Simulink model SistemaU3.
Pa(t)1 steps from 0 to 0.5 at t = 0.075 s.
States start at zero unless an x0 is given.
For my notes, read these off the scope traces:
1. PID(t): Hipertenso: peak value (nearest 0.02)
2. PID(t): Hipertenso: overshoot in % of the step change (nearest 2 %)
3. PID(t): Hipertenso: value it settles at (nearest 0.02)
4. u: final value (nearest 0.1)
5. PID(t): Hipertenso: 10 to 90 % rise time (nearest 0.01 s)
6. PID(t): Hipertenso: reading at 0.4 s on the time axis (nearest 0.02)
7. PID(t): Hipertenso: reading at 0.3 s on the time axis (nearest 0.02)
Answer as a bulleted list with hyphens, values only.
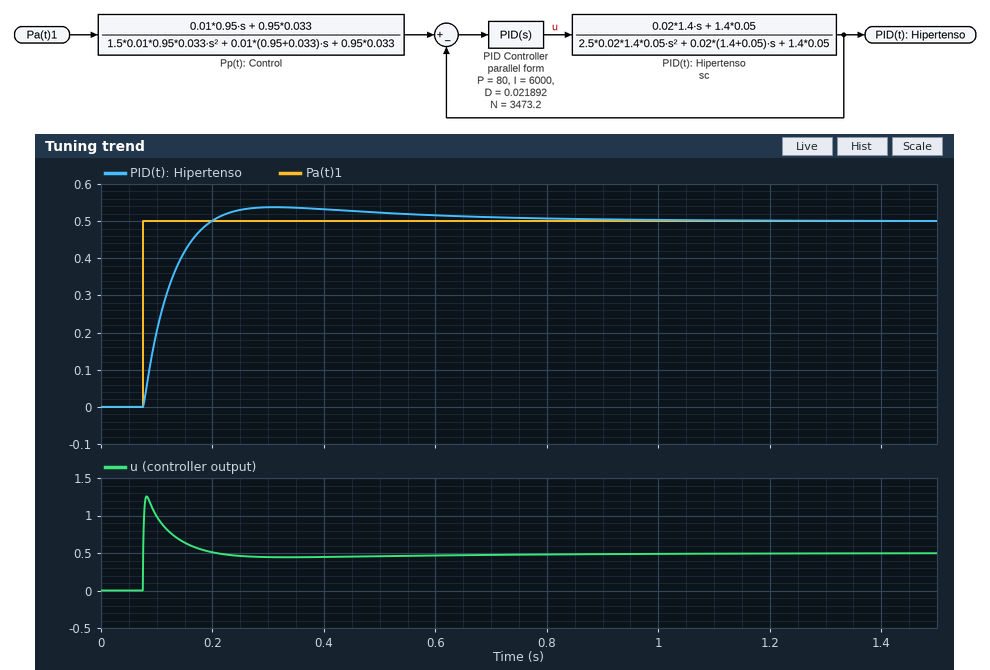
- 0.54
- 8 %
- 0.50
- 0.5
- 0.08 s
- 0.54
- 0.54
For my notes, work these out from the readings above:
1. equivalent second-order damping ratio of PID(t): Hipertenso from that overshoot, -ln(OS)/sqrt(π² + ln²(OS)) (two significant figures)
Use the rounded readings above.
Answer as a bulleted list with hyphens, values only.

- 0.63
